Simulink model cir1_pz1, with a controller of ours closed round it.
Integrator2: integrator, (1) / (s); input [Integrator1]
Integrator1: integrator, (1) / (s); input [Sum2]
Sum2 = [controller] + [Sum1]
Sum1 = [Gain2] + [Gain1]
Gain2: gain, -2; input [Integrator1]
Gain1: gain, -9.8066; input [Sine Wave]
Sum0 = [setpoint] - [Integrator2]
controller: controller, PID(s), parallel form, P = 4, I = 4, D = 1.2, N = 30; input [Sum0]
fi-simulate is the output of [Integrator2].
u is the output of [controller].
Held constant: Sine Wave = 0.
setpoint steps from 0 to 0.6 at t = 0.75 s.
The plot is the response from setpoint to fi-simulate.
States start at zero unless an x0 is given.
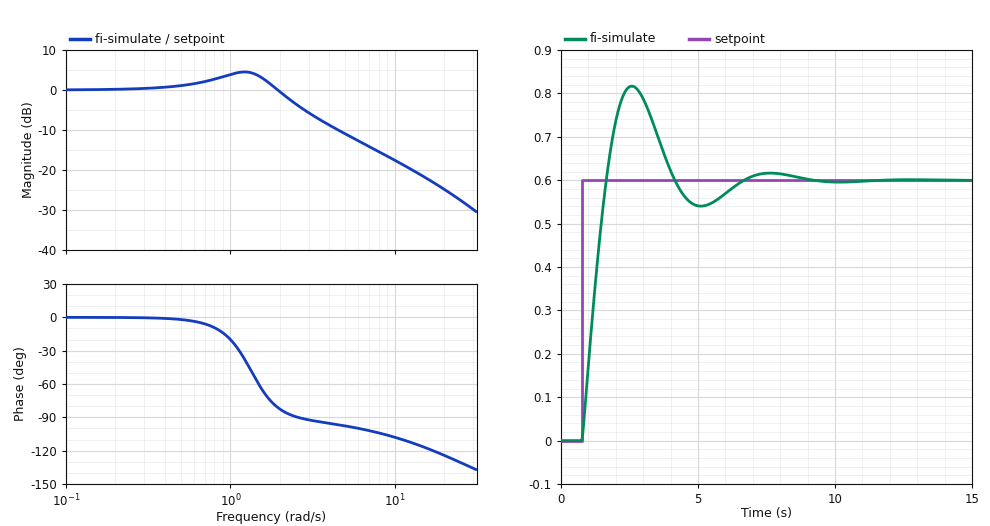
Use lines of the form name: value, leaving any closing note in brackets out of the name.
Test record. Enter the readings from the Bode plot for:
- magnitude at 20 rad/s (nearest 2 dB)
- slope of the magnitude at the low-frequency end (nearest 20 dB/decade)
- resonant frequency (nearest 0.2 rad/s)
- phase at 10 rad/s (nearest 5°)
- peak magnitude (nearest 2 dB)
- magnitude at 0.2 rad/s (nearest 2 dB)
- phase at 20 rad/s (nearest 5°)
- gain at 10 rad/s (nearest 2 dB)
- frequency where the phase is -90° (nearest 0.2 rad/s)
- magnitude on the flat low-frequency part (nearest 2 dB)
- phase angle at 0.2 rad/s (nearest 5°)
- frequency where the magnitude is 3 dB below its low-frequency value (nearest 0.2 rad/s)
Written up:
magnitude at 20 rad/s: -24 dB
slope of the magnitude at the low-frequency end: 0 dB/decade
resonant frequency: 1.2 rad/s
phase at 10 rad/s: -110°
peak magnitude: 4 dB
magnitude at 0.2 rad/s: 0 dB
phase at 20 rad/s: -125°
gain at 10 rad/s: -18 dB
frequency where the phase is -90°: 2.6 rad/s
magnitude on the flat low-frequency part: 0 dB
phase angle at 0.2 rad/s: 0°
frequency where the magnitude is 3 dB below its low-frequency value: 2.4 rad/s
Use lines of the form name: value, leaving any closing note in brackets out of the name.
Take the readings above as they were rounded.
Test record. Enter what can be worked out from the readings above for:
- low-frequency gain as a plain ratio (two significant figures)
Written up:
low-frequency gain as a plain ratio: 1.0
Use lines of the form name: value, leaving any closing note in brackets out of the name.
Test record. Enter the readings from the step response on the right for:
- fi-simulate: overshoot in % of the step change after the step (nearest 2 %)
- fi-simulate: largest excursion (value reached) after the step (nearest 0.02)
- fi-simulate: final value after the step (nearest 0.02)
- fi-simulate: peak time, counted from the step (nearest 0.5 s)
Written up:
fi-simulate: overshoot in % of the step change after the step: 36 %
fi-simulate: largest excursion (value reached) after the step: 0.82
fi-simulate: final value after the step: 0.60
fi-simulate: peak time, counted from the step: 2.0 s
